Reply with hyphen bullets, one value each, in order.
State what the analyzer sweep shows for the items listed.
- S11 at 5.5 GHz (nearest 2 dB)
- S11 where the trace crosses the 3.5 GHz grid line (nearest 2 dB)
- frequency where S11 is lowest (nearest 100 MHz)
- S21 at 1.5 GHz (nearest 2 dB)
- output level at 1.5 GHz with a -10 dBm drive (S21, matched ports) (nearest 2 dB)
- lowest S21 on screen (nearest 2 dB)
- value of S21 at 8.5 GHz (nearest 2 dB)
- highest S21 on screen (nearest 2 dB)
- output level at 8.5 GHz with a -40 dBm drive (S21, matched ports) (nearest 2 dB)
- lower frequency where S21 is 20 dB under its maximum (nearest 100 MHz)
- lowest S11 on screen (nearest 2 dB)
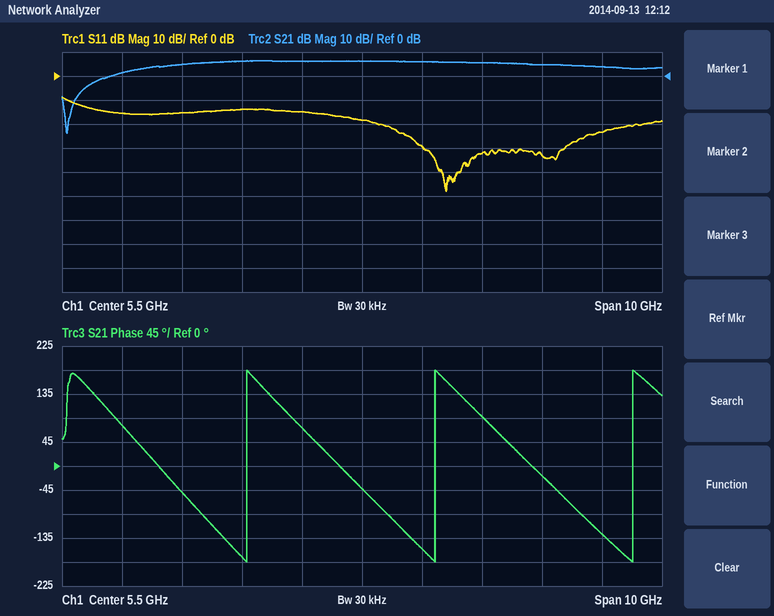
- -18 dB
- -14 dB
- 6.9 GHz
- 2 dB
- -8 dBm
- -24 dB
- 4 dB
- 6 dB
- -36 dBm
- 700 MHz
- -48 dB
